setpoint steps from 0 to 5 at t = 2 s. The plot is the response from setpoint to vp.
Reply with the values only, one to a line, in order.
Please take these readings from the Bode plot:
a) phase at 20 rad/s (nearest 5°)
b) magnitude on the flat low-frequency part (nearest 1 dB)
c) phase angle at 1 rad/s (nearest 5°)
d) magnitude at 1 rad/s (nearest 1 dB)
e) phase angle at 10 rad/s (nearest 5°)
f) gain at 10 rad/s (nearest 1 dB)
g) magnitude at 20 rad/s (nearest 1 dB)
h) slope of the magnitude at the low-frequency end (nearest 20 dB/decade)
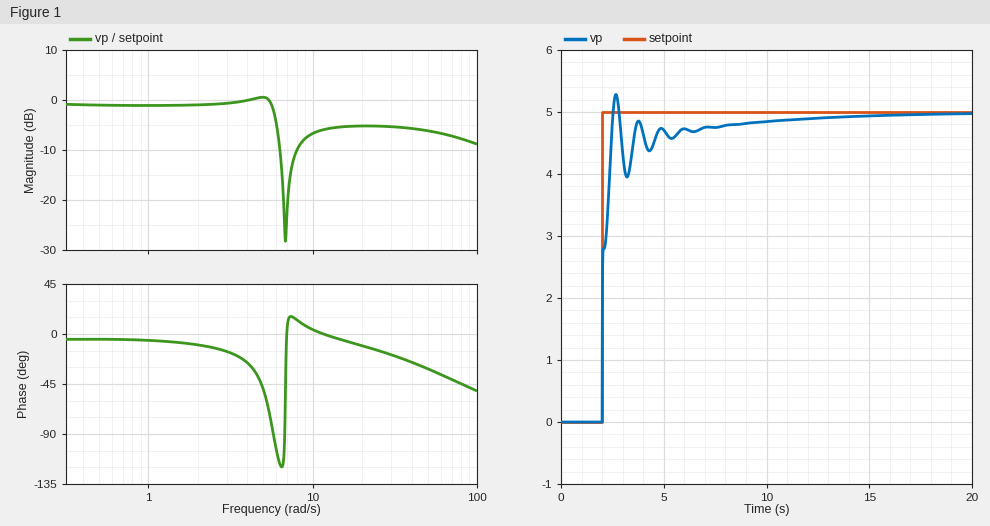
-10°
-1 dB
-5°
-1 dB
5°
-7 dB
-5 dB
0 dB/decade
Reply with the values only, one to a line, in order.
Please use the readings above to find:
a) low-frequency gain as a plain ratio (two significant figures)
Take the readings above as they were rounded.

0.89
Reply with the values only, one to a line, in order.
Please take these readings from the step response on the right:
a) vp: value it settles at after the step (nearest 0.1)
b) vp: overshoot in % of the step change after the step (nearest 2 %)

5.0
6 %
